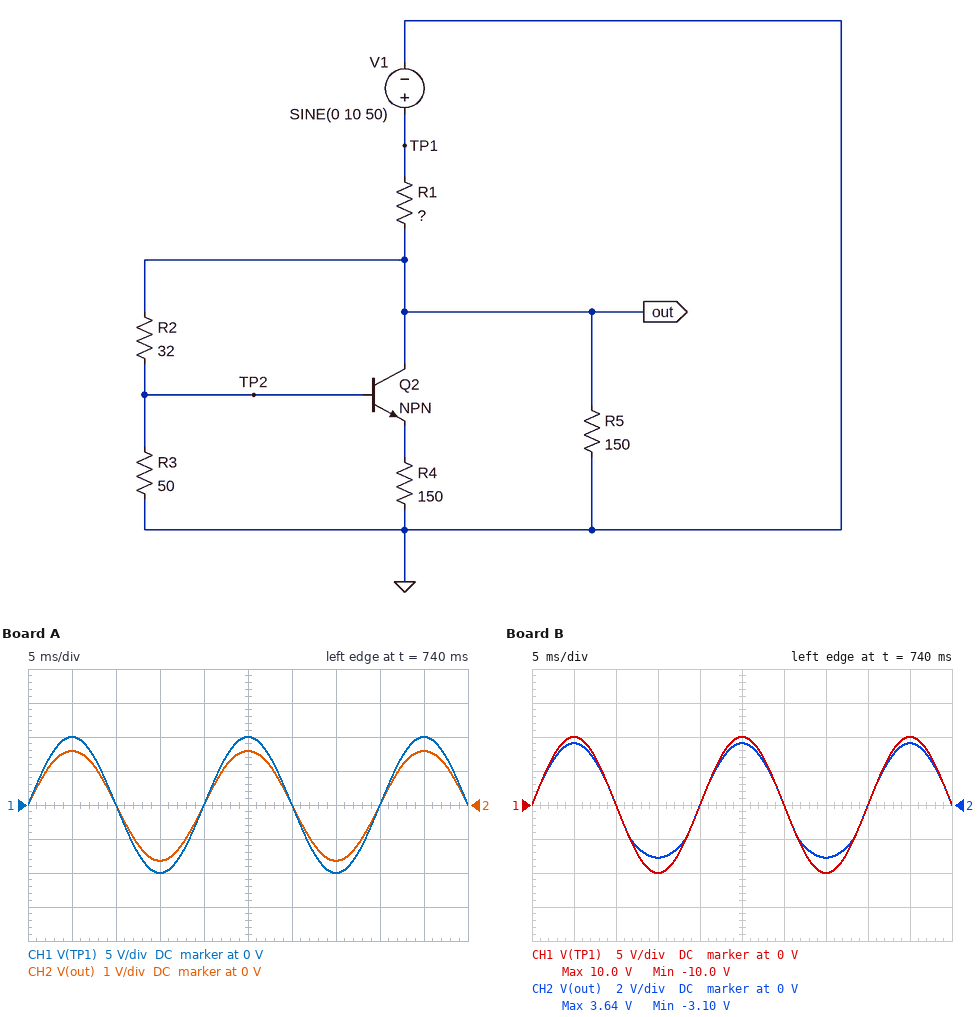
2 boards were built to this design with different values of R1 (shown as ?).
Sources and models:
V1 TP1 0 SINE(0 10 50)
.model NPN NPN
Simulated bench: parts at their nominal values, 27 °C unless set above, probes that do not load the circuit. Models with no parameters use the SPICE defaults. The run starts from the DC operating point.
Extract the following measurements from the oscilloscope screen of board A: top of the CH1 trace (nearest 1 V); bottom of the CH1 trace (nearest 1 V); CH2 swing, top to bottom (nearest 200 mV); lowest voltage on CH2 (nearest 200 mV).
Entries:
10 V
-10 V
3.2 V
-1.6 V
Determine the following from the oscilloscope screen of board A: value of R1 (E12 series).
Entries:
270 Ω
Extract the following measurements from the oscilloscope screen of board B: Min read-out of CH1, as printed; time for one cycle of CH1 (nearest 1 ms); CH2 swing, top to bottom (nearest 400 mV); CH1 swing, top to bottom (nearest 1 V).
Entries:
-10.0 V
20 ms
6.8 V
20 V
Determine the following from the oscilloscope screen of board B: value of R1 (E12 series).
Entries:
82 Ω
